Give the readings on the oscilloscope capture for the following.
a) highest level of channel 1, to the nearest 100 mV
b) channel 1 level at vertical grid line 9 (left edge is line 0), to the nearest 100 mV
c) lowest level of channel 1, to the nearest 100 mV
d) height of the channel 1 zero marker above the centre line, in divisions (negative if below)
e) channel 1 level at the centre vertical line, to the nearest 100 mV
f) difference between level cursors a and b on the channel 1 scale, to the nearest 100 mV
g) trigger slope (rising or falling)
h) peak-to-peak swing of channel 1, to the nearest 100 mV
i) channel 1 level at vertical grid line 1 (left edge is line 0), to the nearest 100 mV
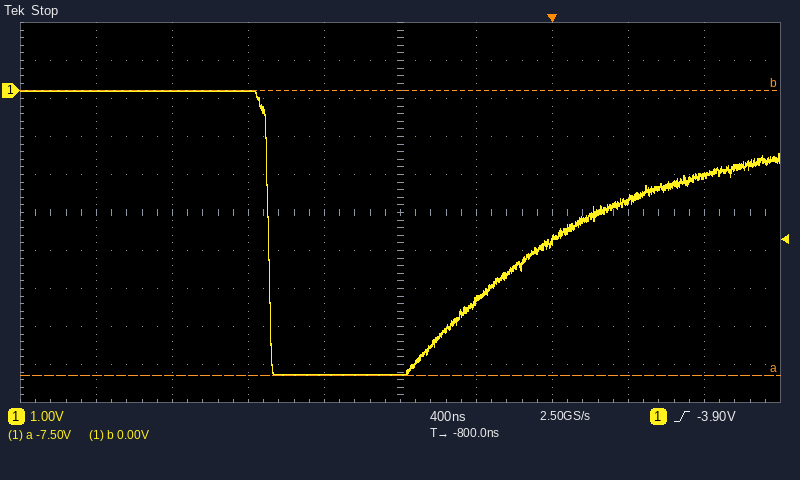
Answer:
0.0 V
-2.2 V
-7.5 V
+3.2 div
-7.5 V
7.5 V
rising
7.5 V
0.0 V
